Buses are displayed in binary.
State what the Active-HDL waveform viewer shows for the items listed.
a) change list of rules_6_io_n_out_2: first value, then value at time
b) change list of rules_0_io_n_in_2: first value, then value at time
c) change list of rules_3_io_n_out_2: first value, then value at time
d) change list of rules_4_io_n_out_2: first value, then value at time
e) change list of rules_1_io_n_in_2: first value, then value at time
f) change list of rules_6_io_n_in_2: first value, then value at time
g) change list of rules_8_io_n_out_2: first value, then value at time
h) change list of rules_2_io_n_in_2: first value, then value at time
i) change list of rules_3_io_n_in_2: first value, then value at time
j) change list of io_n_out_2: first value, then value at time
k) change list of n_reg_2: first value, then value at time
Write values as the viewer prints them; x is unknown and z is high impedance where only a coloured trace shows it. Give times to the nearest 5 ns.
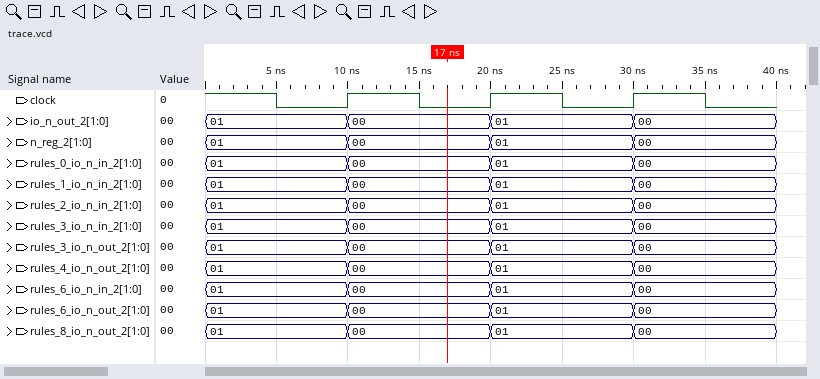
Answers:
01, 00 at 10 ns, 01 at 20 ns, 00 at 30 ns
01, 00 at 10 ns, 01 at 20 ns, 00 at 30 ns
01, 00 at 10 ns, 01 at 20 ns, 00 at 30 ns
01, 00 at 10 ns, 01 at 20 ns, 00 at 30 ns
01, 00 at 10 ns, 01 at 20 ns, 00 at 30 ns
01, 00 at 10 ns, 01 at 20 ns, 00 at 30 ns
01, 00 at 10 ns, 01 at 20 ns, 00 at 30 ns
01, 00 at 10 ns, 01 at 20 ns, 00 at 30 ns
01, 00 at 10 ns, 01 at 20 ns, 00 at 30 ns
01, 00 at 10 ns, 01 at 20 ns, 00 at 30 ns
01, 00 at 10 ns, 01 at 20 ns, 00 at 30 ns
